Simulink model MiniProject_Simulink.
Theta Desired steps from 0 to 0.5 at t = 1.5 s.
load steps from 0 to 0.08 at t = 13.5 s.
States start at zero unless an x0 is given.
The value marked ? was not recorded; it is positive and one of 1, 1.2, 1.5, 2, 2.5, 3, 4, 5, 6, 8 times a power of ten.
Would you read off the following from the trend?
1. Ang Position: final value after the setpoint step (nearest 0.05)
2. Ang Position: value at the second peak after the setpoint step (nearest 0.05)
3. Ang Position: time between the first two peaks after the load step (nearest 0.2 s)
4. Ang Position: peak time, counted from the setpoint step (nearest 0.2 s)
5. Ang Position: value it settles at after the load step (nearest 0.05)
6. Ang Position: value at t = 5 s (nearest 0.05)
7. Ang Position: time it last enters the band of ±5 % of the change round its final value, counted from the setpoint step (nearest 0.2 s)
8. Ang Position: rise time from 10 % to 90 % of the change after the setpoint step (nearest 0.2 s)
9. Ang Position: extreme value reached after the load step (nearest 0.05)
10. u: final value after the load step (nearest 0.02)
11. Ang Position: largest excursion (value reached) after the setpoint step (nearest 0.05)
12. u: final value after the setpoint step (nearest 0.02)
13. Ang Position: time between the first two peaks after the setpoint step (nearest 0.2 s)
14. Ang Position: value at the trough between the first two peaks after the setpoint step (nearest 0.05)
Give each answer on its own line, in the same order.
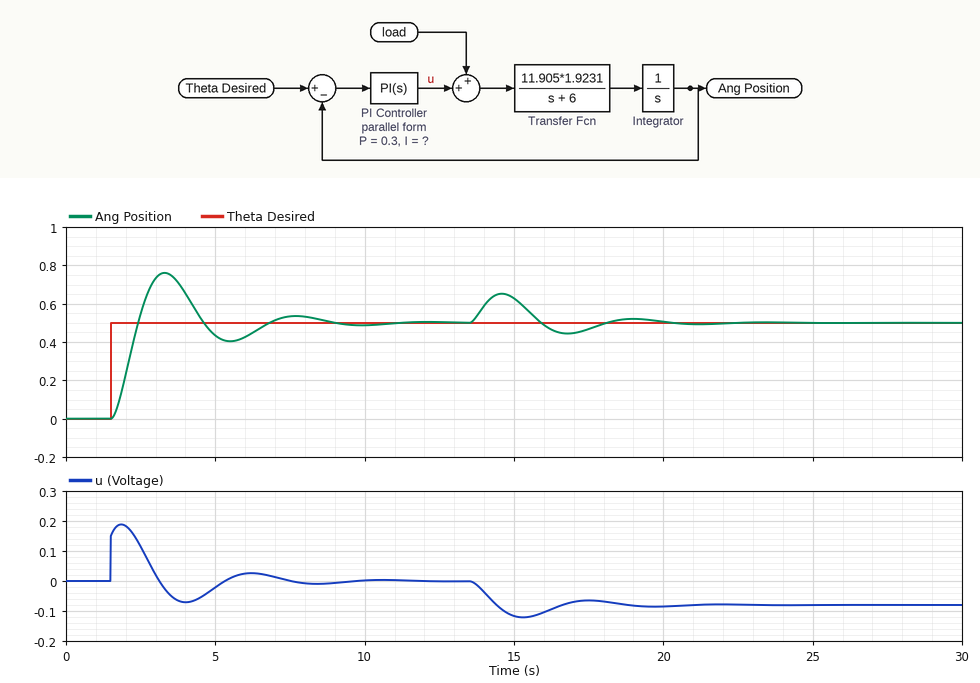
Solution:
0.50
0.55
4.4 s
1.8 s
0.50
0.45
6.8 s
0.6 s
0.65
-0.08
0.75
0.00
4.4 s
0.40
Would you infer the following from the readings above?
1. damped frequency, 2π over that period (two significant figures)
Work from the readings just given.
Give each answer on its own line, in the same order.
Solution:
1.4 rad/s
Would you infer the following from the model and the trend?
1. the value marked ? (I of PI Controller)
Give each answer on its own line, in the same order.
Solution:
0.5
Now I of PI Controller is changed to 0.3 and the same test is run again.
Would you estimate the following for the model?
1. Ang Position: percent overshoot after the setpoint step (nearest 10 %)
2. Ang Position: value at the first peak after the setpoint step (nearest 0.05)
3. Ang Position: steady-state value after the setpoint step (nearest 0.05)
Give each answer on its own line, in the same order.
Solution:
40 %
0.70
0.50
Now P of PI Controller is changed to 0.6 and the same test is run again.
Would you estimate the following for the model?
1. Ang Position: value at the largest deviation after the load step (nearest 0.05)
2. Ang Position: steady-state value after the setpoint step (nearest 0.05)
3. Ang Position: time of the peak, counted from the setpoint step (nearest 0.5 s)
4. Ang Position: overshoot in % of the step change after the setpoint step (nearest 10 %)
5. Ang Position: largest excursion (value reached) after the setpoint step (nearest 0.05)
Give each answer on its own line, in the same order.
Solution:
0.60
0.50
1.5 s
30 %
0.65
